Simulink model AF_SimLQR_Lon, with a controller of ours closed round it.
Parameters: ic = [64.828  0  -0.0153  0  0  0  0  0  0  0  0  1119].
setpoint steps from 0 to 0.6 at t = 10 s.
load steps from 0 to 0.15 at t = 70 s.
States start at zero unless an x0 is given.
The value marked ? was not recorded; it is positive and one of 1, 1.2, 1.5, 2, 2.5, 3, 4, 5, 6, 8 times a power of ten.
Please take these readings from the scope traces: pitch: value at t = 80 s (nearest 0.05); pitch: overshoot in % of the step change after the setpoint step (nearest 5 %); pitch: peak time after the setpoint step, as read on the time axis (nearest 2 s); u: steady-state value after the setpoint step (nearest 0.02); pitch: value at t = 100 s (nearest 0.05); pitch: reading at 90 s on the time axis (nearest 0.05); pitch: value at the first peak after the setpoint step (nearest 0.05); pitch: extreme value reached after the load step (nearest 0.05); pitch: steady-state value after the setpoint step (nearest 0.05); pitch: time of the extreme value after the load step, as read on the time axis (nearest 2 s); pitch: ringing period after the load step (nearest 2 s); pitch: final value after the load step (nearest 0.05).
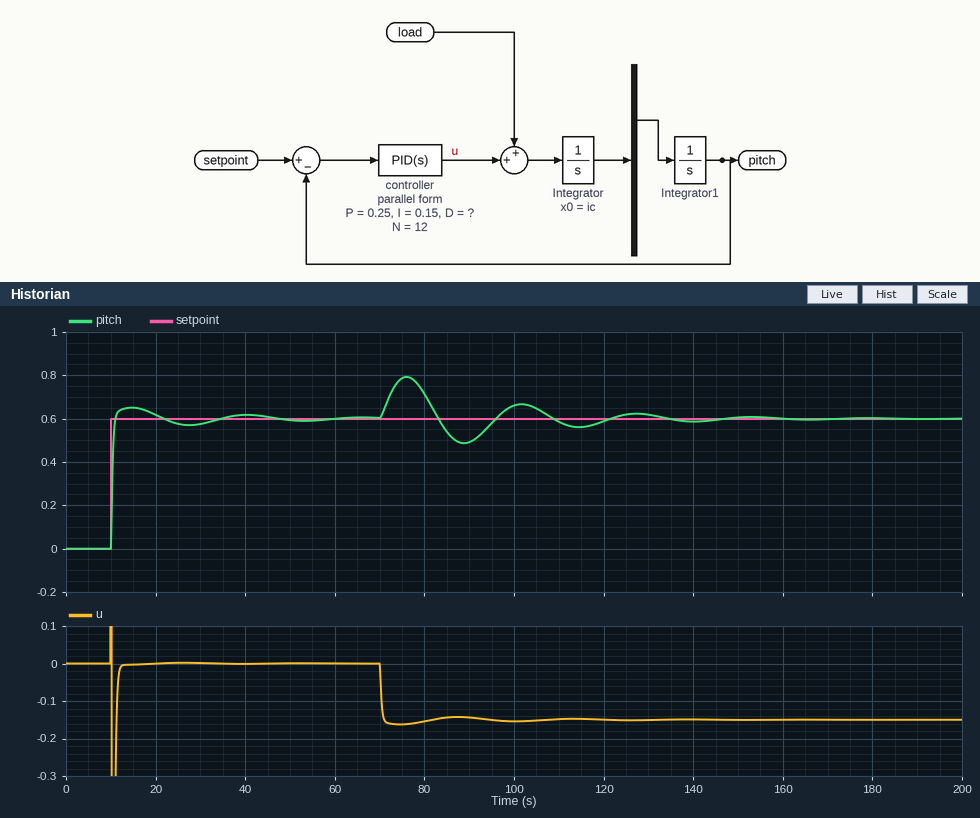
0.70
10 %
14 s
0.00
0.65
0.50
0.65
0.80
0.60
76 s
26 s
0.60
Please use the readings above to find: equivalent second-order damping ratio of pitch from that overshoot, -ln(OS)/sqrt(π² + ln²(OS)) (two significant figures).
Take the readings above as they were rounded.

0.59
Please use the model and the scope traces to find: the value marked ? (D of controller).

2.5
